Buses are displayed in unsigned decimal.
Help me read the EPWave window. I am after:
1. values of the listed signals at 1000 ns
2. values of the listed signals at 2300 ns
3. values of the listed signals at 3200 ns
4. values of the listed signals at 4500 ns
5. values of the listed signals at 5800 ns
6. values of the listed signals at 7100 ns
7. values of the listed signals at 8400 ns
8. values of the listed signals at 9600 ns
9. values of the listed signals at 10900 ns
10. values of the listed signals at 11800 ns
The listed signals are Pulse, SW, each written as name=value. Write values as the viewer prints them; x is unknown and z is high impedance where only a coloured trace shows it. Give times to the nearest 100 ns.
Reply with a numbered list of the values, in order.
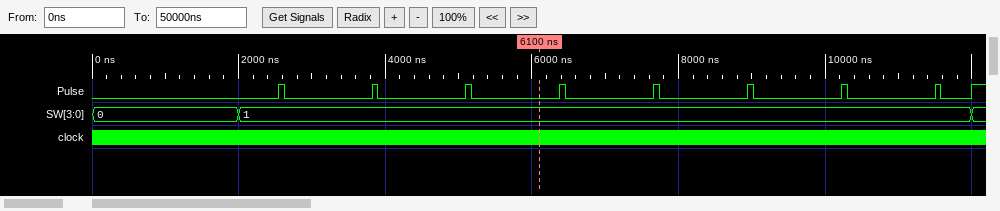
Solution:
1. Pulse=0, SW=0
2. Pulse=0, SW=1
3. Pulse=0, SW=1
4. Pulse=0, SW=1
5. Pulse=0, SW=1
6. Pulse=0, SW=1
7. Pulse=0, SW=1
8. Pulse=0, SW=1
9. Pulse=0, SW=1
10. Pulse=0, SW=1
